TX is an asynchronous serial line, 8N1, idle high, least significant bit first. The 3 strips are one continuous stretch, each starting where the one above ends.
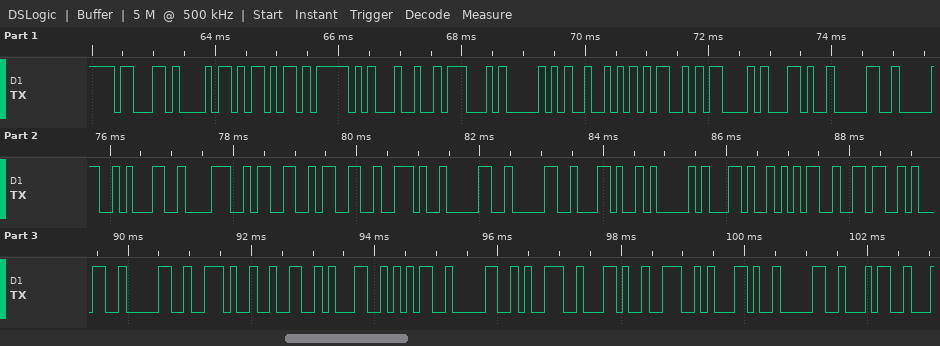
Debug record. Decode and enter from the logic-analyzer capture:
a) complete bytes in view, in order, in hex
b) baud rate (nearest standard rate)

0x63 0x68 0x6B 0x5F 0x24 0x47 0x50 0x52 0x4D 0x43 0x2C 0x30 0x30 0x31 0x38 0x33 0x33 0x2E 0x30 0x30 0x2C 0x41 0x2C 0x35 0x36 0x31 0x30 0x2E 0x32 0x31 0x35 0x30 0x39 0x2C 0x4E 0x2C 0x30 0x34
9600 baud
